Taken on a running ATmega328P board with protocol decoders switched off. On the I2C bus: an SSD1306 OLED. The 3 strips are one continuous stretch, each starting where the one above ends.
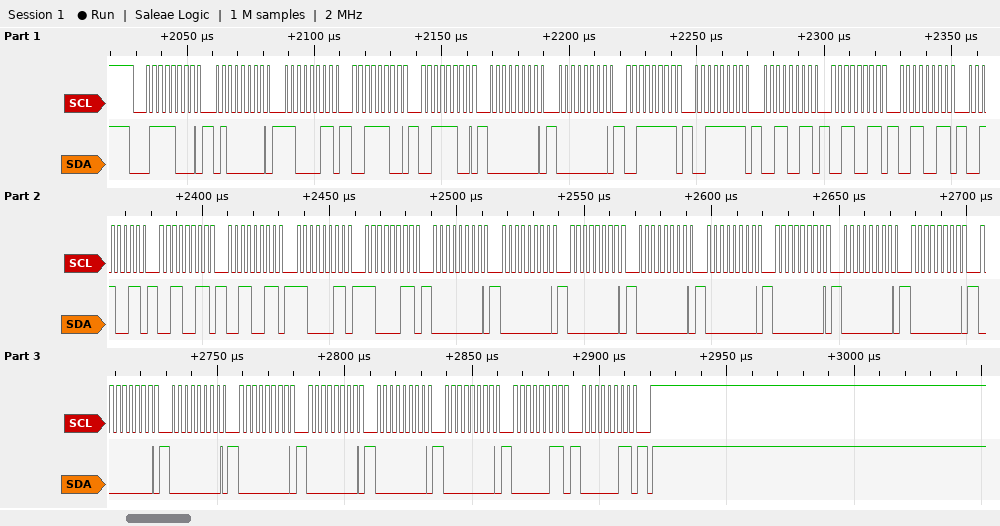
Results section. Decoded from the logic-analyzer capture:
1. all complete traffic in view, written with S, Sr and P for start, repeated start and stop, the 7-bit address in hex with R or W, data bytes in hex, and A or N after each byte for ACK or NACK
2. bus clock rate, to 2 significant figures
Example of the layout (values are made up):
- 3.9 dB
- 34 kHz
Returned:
- S 3CW A 40 A C3 A 3C A 3C A 00 A 00 A 3F A 3F A 33 A 33 A 33 A 33 A 33 A 33 A C3 A C3 A 00 A 00 A 00 A 00 A 00 A 00 A 00 A 00 A 00 A 00 A 00 A 00 A 00 A 00 A 03 A 03 A P
- 400 kHz
